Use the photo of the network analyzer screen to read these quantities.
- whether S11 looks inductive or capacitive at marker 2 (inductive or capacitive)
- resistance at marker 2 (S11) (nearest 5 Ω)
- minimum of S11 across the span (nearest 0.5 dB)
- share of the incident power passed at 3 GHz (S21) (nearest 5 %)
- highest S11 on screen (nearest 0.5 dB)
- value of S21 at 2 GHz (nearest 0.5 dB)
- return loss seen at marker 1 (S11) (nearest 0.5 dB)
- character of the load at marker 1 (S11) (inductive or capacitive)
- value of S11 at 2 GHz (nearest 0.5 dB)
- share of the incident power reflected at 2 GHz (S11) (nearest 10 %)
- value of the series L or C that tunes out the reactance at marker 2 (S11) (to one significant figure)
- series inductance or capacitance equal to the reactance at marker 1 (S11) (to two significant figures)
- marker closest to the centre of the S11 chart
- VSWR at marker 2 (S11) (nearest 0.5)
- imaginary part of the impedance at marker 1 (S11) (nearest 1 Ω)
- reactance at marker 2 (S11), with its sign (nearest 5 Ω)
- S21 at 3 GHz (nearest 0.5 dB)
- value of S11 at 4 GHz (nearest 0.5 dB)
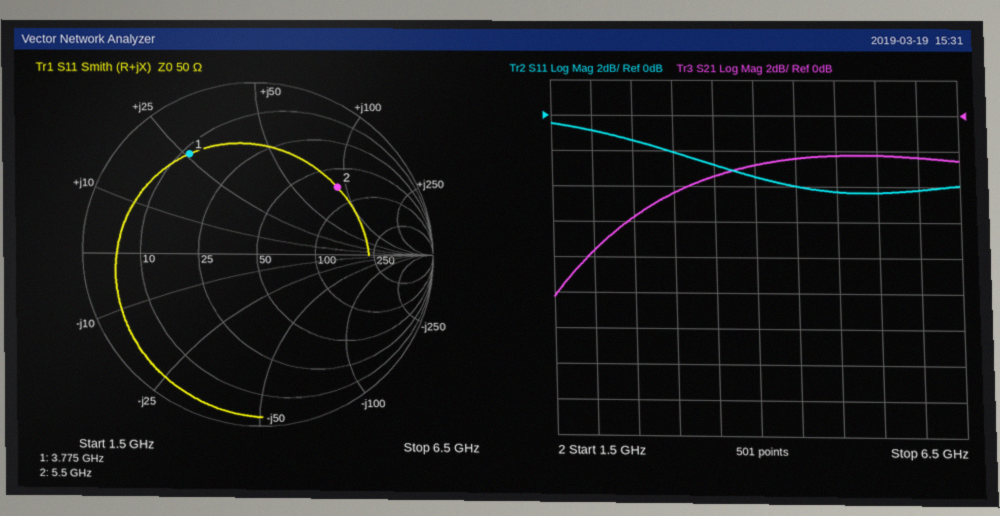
inductive
70 Ω
-4.5 dB
35 %
-0.5 dB
-7.5 dB
3.0 dB
inductive
-1.0 dB
80 %
300 fF
1.1 nH
marker 2
4.0
+26 Ω
+90 Ω
-4.5 dB
-3.5 dB
